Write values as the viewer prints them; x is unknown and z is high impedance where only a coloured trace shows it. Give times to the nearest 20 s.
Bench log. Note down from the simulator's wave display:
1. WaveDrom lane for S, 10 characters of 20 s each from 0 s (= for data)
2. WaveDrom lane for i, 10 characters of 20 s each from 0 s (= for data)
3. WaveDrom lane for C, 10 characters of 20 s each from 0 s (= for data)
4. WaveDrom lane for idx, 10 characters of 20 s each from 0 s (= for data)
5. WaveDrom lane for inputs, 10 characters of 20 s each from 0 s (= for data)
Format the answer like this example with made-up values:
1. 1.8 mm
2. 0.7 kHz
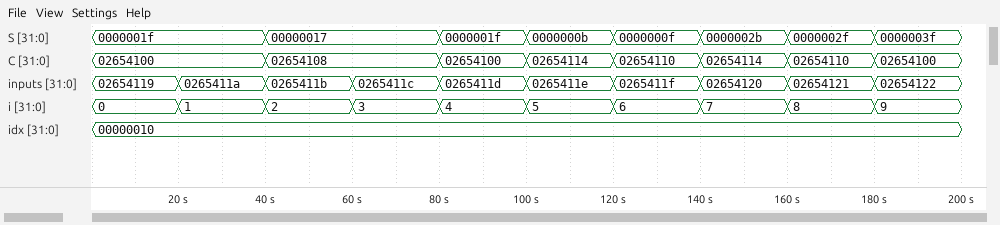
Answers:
1. {name: 'S', wave: '=.=.======', data: '0000001f 00000017 0000001f 0000000b 0000000f 0000002b 0000002f 0000003f'}
2. {name: 'i', wave: '==========', data: '0 1 2 3 4 5 6 7 8 9'}
3. {name: 'C', wave: '=.=.======', data: '02654100 02654108 02654100 02654114 02654110 02654114 02654110 02654100'}
4. {name: 'idx', wave: '=.........', data: '00000010'}
5. {name: 'inputs', wave: '==========', data: '02654119 0265411a 0265411b 0265411c 0265411d 0265411e 0265411f 02654120 02654121 02654122'}
